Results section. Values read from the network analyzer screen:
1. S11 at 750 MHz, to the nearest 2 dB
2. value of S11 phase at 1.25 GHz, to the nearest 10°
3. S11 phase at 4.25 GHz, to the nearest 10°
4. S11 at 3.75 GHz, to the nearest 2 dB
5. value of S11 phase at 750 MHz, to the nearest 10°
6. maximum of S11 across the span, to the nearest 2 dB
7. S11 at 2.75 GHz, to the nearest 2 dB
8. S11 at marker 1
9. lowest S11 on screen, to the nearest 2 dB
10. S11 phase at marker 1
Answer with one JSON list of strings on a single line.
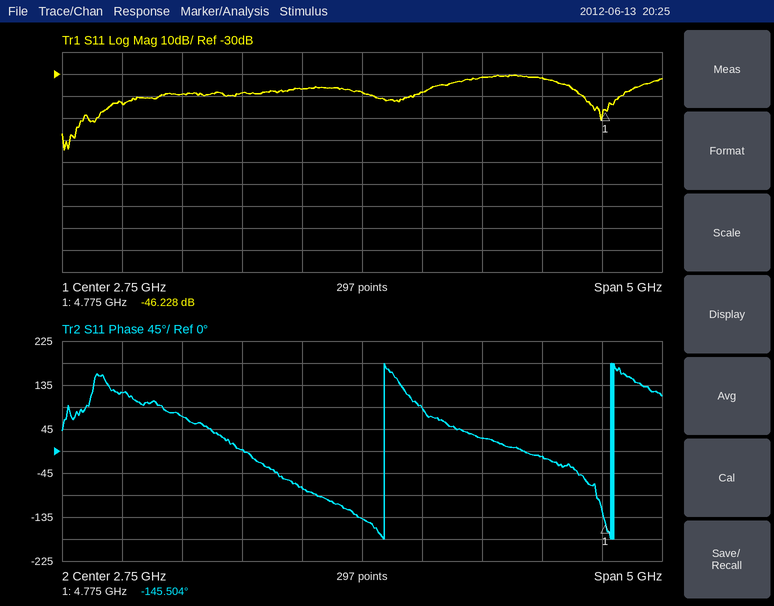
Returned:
["-44 dB", "70°", "-10°", "-32 dB", "120°", "-30 dB", "-38 dB", "-46.228 dB", "-64 dB", "-145.504°"]
